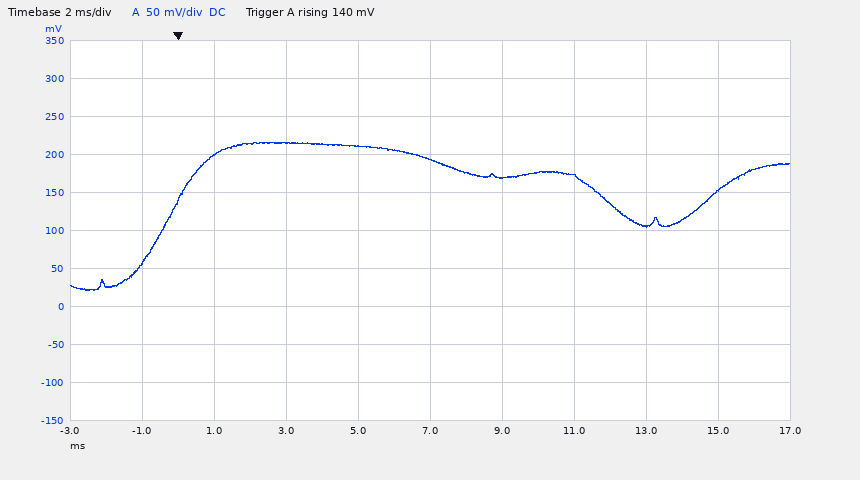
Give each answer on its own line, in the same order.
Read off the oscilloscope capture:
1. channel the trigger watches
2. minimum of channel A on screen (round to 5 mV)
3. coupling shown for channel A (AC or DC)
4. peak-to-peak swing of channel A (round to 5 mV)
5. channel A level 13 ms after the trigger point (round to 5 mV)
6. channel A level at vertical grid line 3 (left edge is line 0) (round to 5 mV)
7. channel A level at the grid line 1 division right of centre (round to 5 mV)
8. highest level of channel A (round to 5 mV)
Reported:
channel A
20 mV
DC
195 mV
105 mV
215 mV
170 mV
215 mV
